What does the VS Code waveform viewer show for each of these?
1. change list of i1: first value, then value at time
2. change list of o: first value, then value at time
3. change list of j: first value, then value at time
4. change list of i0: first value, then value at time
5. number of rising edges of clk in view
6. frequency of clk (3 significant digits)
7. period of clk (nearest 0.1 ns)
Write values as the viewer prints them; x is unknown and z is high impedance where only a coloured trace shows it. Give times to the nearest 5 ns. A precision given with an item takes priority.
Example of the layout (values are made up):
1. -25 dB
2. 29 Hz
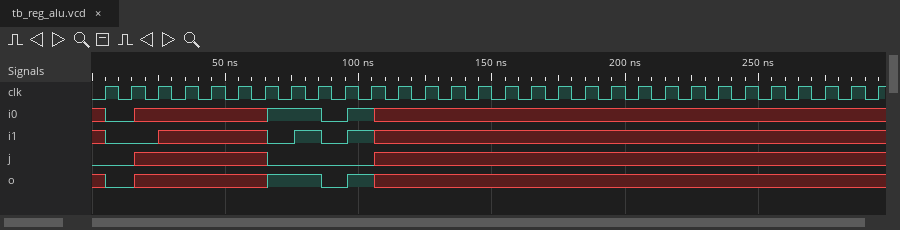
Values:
1. x, 0 at 5 ns, x at 25 ns, 0 at 65 ns, 1 at 75 ns, 0 at 85 ns, 1 at 95 ns, x at 105 ns
2. x, 0 at 5 ns, x at 15 ns, 1 at 65 ns, 0 at 85 ns, 1 at 95 ns, x at 105 ns
3. 0, x at 15 ns, 0 at 65 ns, x at 105 ns
4. x, 0 at 5 ns, x at 15 ns, 1 at 65 ns, 0 at 85 ns, 1 at 95 ns, x at 105 ns
5. 30
6. 100 MHz
7. 10 ns
